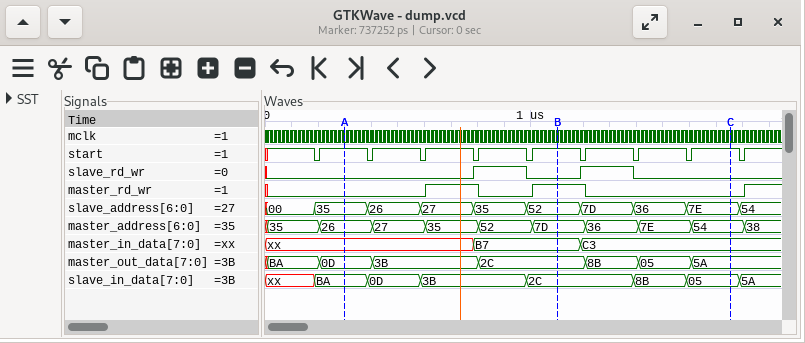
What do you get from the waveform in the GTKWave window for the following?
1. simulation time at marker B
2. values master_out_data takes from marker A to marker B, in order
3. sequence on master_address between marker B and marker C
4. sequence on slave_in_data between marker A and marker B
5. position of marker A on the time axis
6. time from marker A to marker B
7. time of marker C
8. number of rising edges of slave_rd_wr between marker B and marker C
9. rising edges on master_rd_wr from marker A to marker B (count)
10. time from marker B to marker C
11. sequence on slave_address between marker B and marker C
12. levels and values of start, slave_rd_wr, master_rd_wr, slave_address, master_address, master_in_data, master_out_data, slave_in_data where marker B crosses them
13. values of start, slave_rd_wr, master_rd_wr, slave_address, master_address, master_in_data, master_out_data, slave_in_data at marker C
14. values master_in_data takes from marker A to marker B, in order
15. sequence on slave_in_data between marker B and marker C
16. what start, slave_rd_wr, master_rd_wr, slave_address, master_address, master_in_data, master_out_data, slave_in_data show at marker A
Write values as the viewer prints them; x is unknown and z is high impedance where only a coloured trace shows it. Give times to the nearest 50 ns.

1100 ns
0D, 3B, 2C
7D, 36, 7E, 54
BA, 0D, 3B, 2C
300 ns
800 ns
1750 ns
1
2
650 ns
52, 7D, 36, 7E
start=1, slave_rd_wr=0, master_rd_wr=1, slave_address=52, master_address=7D, master_in_data=B7, master_out_data=2C, slave_in_data=2C
start=1, slave_rd_wr=0, master_rd_wr=0, slave_address=7E, master_address=54, master_in_data=C3, master_out_data=5A, slave_in_data=05
xx, B7
2C, 8B, 05
start=1, slave_rd_wr=0, master_rd_wr=0, slave_address=35, master_address=26, master_in_data=xx, master_out_data=0D, slave_in_data=BA
